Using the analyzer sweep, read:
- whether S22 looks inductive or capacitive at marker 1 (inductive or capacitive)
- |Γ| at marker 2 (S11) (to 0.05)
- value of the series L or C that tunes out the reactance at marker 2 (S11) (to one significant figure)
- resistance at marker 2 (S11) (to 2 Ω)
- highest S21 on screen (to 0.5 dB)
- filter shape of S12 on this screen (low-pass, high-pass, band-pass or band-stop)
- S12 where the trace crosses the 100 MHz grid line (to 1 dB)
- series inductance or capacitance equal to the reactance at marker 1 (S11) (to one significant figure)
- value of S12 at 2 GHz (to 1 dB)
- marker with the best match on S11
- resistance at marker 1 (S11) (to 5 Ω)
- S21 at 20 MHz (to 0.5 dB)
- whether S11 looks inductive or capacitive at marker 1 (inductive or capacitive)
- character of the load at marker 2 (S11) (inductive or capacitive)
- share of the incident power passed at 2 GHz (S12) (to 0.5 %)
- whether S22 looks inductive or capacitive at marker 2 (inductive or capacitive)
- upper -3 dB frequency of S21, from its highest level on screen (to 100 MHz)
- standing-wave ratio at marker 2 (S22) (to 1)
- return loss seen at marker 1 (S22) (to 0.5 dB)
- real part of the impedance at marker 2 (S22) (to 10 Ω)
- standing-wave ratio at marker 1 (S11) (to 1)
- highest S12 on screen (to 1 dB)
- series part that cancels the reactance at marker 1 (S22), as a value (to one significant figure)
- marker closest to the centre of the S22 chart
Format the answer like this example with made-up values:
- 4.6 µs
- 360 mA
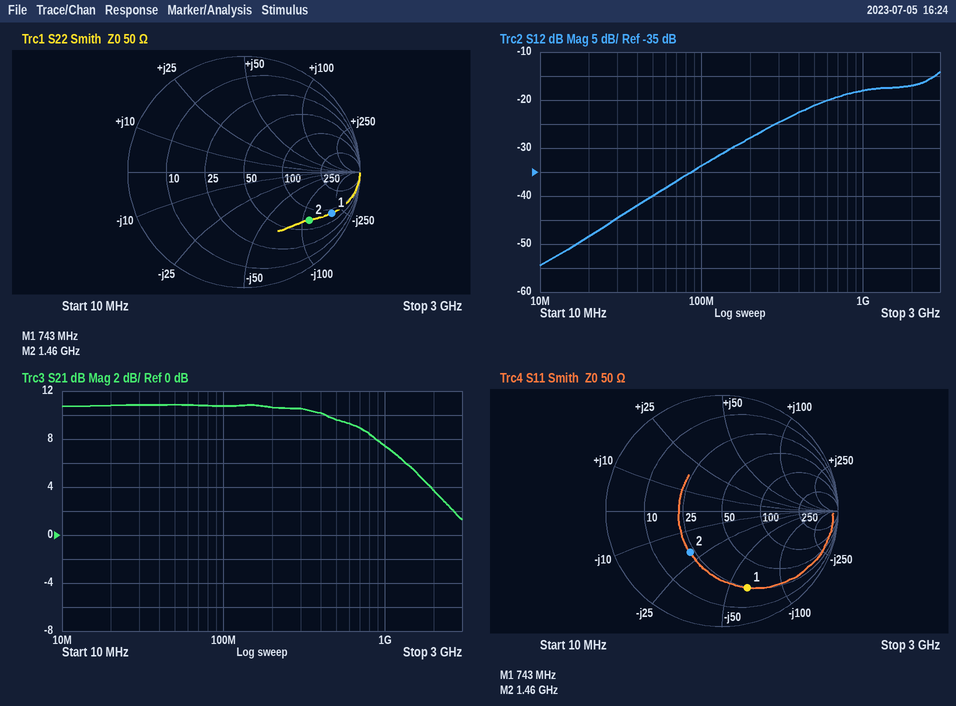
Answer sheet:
- capacitive
- 0.45
- 2 nH
- 22 Ω
- 11.0 dB
- high-pass
- -34 dB
- 3 pF
- -17 dB
- marker 2
- 25 Ω
- 11.0 dB
- capacitive
- capacitive
- 2.0 %
- capacitive
- 900 MHz
- 6
- 1.5 dB
- 70 Ω
- 6
- -14 dB
- 40 nH
- marker 2
